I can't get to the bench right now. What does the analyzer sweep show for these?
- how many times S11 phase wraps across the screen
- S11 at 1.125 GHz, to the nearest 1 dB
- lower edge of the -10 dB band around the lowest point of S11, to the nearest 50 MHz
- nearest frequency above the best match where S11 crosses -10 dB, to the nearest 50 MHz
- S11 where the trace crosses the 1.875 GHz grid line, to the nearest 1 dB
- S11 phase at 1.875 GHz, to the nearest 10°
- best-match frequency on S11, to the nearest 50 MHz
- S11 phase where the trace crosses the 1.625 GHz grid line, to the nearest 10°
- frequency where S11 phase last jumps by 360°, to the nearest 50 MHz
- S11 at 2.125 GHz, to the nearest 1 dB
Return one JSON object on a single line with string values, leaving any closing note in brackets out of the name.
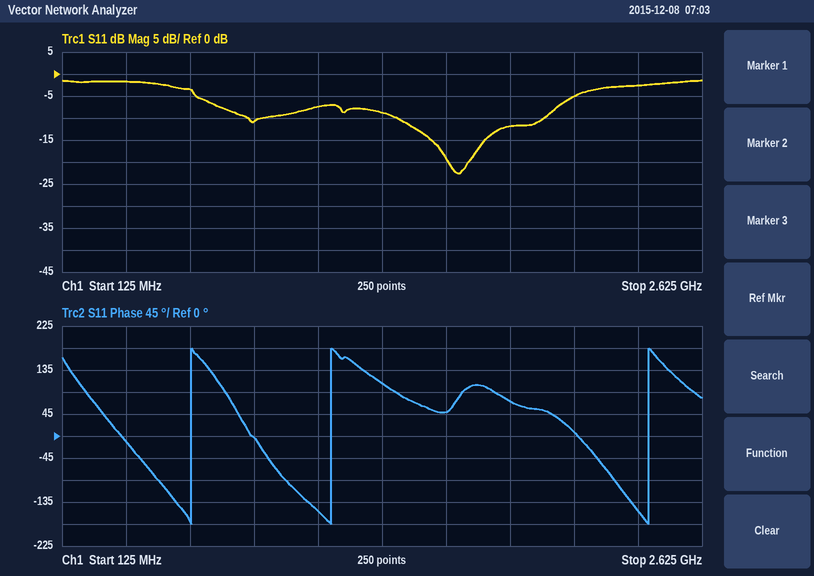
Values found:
{"how many times S11 phase wraps across the screen": "3", "S11 at 1.125 GHz, to the nearest 1 dB": "-7 dB", "lower edge of the -10 dB band around the lowest point of S11, to the nearest 50 MHz": "1.45 GHz", "nearest frequency above the best match where S11 crosses -10 dB, to the nearest 50 MHz": "2.00 GHz", "S11 where the trace crosses the 1.875 GHz grid line, to the nearest 1 dB": "-12 dB", "S11 phase at 1.875 GHz, to the nearest 10°": "70°", "best-match frequency on S11, to the nearest 50 MHz": "1.65 GHz", "S11 phase where the trace crosses the 1.625 GHz grid line, to the nearest 10°": "50°", "frequency where S11 phase last jumps by 360°, to the nearest 50 MHz": "2.40 GHz", "S11 at 2.125 GHz, to the nearest 1 dB": "-5 dB"}
